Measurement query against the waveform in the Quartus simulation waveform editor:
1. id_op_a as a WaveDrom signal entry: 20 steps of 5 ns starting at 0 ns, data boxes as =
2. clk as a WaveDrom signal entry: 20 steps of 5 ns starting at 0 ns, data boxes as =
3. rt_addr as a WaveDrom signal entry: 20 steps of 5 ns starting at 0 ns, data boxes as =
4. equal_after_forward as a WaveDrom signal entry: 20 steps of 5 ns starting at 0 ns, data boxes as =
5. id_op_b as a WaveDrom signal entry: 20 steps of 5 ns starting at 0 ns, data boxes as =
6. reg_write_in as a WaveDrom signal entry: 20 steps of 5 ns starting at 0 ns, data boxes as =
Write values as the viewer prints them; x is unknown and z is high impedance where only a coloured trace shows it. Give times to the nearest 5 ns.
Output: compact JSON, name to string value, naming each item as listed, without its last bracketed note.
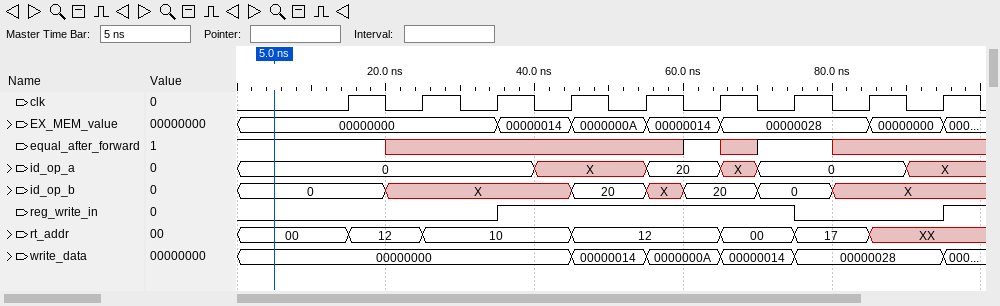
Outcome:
{"id_op_a as a WaveDrom signal entry: 20 steps of 5 ns starting at 0 ns, data boxes as =": "{name: 'id_op_a', wave: '=.......x..=.x=...x.', data: '0 20 0'}", "clk as a WaveDrom signal entry: 20 steps of 5 ns starting at 0 ns, data boxes as =": "{name: 'clk', wave: '0..10101010101010101'}", "rt_addr as a WaveDrom signal entry: 20 steps of 5 ns starting at 0 ns, data boxes as =": "{name: 'rt_addr', wave: '=..=.=...=...=.=.x..', data: '00 12 10 12 00 17'}", "equal_after_forward as a WaveDrom signal entry: 20 steps of 5 ns starting at 0 ns, data boxes as =": "{name: 'equal_after_forward', wave: '1...x.......1x1.x...'}", "id_op_b as a WaveDrom signal entry: 20 steps of 5 ns starting at 0 ns, data boxes as =": "{name: 'id_op_b', wave: '=...x....=.x=.=.x...', data: '0 20 20 0'}", "reg_write_in as a WaveDrom signal entry: 20 steps of 5 ns starting at 0 ns, data boxes as =": "{name: 'reg_write_in', wave: '0......1.......0...1'}"}
